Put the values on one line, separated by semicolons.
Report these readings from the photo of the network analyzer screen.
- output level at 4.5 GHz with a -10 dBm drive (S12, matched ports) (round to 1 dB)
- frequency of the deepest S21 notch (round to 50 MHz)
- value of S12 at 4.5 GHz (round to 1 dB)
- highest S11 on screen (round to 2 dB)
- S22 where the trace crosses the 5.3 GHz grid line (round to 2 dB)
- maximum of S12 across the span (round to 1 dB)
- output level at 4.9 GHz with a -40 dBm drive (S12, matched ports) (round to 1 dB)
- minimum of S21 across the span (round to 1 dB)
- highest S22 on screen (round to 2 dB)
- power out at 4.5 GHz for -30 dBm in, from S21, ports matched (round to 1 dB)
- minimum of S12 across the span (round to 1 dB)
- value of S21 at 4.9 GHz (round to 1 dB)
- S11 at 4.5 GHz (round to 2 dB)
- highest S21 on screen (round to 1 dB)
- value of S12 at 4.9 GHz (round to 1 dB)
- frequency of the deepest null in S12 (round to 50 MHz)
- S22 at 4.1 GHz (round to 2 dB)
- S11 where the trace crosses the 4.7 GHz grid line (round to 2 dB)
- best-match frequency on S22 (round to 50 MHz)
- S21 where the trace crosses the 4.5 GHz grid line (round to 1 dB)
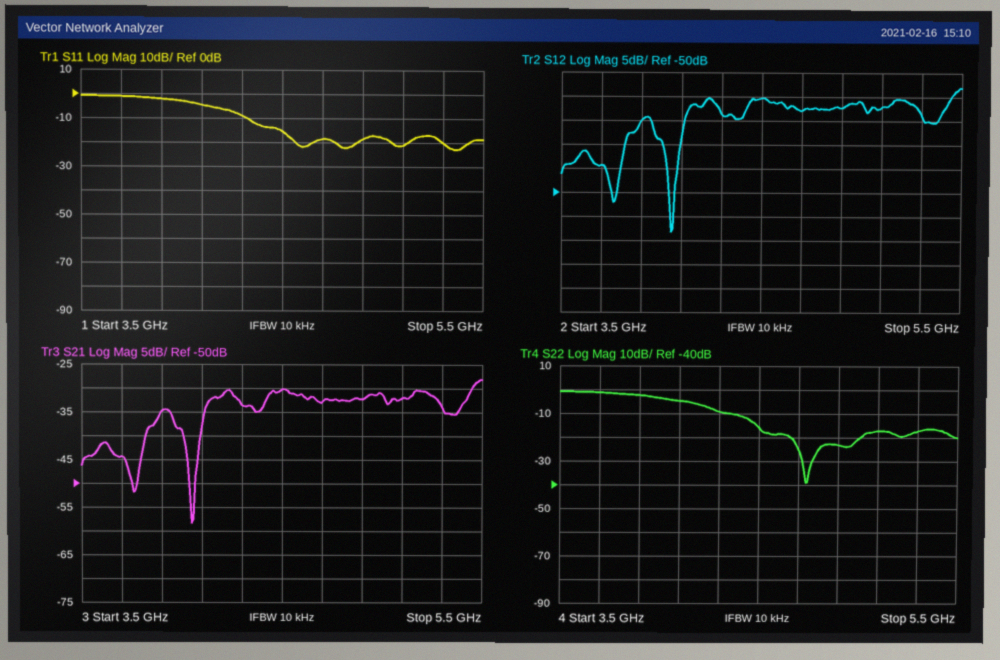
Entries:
-40 dBm; 4.05 GHz; -30 dB; 0 dB; -18 dB; -28 dB; -72 dBm; -58 dB; 0 dB; -60 dBm; -58 dB; -32 dB; -16 dB; -28 dB; -32 dB; 4.05 GHz; -4 dB; -18 dB; 4.75 GHz; -30 dB
